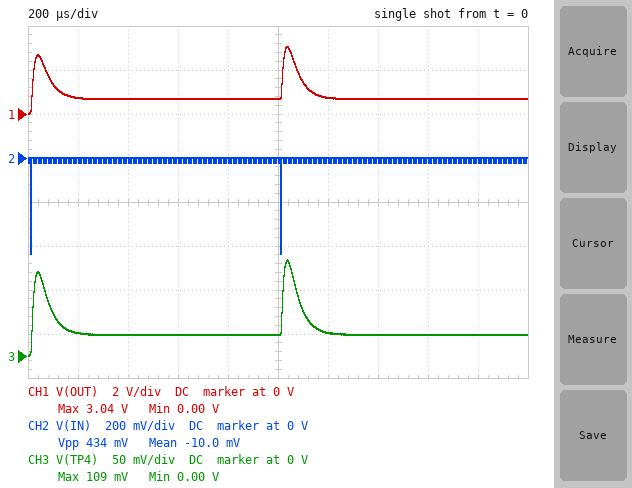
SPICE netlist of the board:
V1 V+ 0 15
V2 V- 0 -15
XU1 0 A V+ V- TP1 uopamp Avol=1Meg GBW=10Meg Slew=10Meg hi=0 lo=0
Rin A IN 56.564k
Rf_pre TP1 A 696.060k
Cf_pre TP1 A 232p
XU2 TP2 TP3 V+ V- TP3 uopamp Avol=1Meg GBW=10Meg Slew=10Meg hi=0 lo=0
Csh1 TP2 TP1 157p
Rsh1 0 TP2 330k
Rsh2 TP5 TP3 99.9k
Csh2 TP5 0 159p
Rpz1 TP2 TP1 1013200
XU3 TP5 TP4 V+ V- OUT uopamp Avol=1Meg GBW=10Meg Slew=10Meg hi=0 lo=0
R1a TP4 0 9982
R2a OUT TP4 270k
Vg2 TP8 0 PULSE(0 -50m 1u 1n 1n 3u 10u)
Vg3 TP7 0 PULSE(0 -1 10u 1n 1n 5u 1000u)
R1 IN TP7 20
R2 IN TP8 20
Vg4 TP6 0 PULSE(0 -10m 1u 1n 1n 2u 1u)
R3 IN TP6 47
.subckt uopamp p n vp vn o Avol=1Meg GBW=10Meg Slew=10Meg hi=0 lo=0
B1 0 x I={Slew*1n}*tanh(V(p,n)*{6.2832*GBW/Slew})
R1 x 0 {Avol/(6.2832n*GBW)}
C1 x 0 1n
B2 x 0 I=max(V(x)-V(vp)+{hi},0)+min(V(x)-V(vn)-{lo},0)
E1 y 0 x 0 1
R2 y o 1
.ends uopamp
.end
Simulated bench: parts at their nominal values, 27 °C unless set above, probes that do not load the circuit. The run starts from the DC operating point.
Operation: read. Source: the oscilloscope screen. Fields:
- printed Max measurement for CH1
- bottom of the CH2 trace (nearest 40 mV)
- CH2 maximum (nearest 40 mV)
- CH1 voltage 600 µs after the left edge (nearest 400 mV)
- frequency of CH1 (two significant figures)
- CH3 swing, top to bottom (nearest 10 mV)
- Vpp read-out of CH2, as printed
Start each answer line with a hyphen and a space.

- 3.04 V
- -440 mV
- 0 V
- 800 mV
- 1.0 kHz
- 110 mV
- 434 mV
